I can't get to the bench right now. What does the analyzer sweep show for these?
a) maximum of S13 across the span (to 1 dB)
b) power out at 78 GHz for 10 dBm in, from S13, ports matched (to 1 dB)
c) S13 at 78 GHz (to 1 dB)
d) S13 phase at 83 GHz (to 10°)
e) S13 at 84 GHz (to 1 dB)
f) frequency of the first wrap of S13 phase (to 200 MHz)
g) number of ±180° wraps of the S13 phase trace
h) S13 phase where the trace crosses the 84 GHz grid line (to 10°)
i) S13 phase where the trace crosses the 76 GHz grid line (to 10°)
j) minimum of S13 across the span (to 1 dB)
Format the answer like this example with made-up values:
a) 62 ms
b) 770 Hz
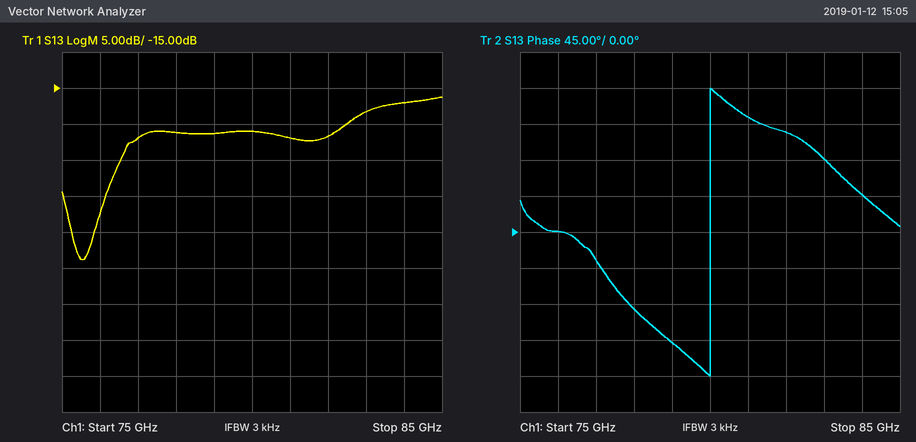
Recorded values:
a) -16 dB
b) -11 dBm
c) -21 dB
d) 90°
e) -17 dB
f) 80.0 GHz
g) 1
h) 50°
i) 0°
j) -39 dB
